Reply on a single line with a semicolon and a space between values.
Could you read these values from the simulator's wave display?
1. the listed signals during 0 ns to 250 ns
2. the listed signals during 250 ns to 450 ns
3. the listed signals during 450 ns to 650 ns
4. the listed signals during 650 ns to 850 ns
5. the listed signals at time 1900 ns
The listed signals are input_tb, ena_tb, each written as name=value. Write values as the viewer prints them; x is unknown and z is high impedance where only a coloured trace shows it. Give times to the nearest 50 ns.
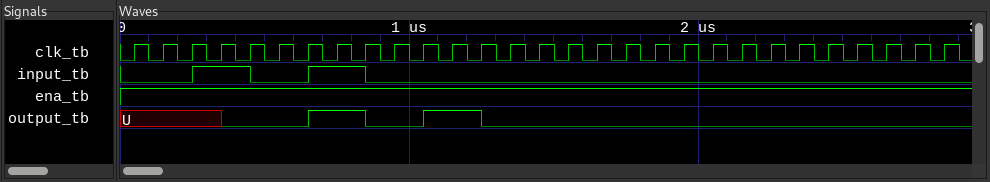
input_tb=0, ena_tb=1; input_tb=1, ena_tb=1; input_tb=0, ena_tb=1; input_tb=1, ena_tb=1; input_tb=0, ena_tb=1
